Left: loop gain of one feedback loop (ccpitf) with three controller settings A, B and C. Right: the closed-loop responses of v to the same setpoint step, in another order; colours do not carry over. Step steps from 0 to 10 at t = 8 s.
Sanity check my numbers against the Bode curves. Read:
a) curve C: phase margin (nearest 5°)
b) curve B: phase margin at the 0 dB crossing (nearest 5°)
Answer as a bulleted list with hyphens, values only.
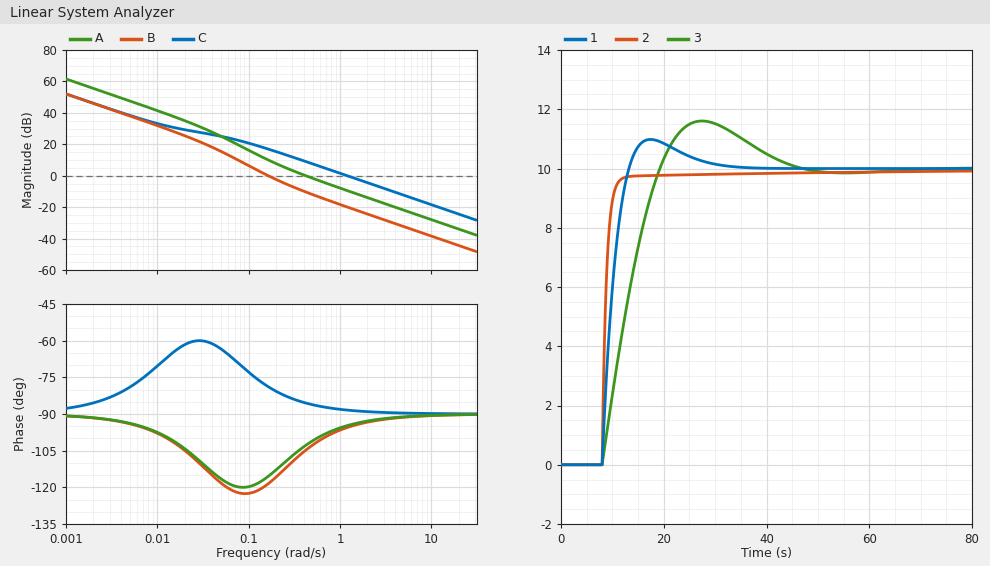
- 90°
- 60°
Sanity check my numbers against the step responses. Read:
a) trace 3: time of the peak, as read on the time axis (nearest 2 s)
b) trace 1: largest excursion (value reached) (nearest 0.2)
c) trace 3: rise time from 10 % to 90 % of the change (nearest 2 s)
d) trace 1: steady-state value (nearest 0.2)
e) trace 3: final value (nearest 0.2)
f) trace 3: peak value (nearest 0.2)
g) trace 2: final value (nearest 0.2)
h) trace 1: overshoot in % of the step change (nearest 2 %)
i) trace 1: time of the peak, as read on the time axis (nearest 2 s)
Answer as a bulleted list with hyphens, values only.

- 28 s
- 11.0
- 8 s
- 10.0
- 10.0
- 11.6
- 10.0
- 10 %
- 18 s
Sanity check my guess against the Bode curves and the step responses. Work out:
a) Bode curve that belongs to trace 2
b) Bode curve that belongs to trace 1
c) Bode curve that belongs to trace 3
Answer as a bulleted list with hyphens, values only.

- C
- A
- B
